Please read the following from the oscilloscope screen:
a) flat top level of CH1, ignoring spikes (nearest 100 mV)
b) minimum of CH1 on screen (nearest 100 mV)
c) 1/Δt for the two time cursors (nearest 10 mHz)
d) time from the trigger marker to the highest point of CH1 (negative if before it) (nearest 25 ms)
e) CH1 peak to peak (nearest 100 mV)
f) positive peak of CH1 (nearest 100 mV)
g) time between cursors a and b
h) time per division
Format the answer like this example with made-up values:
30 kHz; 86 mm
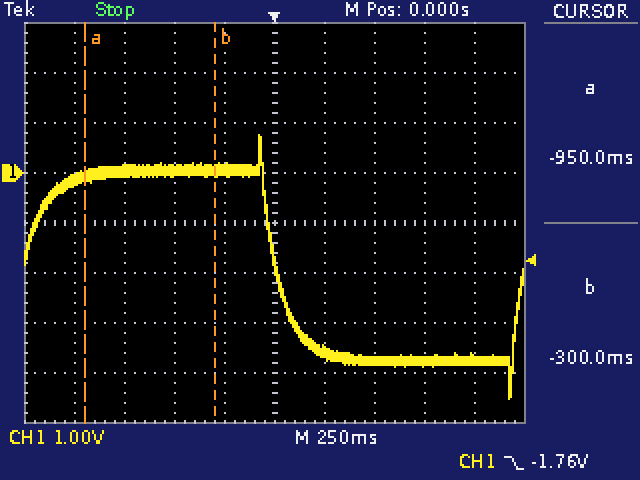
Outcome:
0.0 V; -4.5 V; 1.54 Hz; -75 ms; 5.3 V; 800 mV; 650 ms; 250 ms
